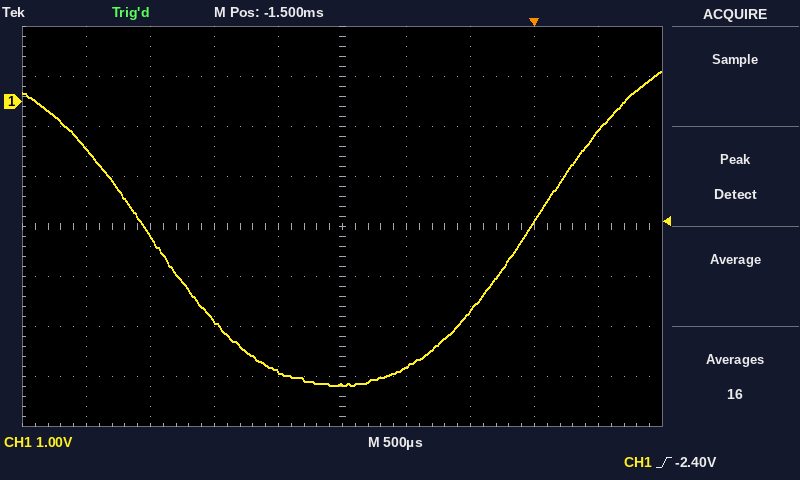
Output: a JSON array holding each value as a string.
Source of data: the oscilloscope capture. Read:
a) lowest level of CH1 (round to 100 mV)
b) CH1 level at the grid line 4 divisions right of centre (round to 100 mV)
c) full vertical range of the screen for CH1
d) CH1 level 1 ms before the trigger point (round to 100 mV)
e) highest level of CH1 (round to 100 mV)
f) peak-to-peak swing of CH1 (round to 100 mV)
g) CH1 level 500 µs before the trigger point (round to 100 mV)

["-5.7 V", "-600 mV", "8 V", "-5.3 V", "600 mV", "6.3 V", "-4.2 V"]
